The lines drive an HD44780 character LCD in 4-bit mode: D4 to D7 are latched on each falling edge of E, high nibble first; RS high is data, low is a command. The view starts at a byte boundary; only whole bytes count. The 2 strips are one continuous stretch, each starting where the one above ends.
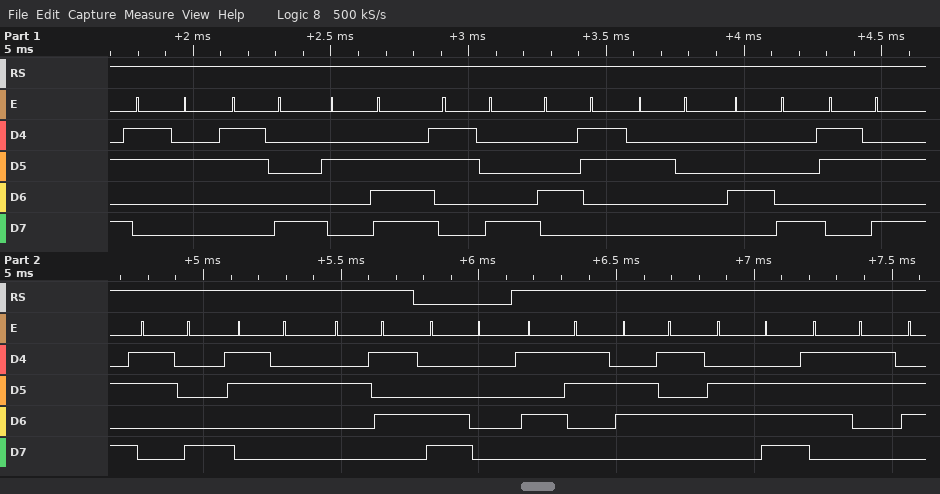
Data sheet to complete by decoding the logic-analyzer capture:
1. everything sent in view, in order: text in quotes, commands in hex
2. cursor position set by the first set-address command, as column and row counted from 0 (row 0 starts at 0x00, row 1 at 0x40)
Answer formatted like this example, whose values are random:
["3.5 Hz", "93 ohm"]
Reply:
["\"28.8C H:82%\" 0xC0 \"Sens\"", "column 0, row 1"]
